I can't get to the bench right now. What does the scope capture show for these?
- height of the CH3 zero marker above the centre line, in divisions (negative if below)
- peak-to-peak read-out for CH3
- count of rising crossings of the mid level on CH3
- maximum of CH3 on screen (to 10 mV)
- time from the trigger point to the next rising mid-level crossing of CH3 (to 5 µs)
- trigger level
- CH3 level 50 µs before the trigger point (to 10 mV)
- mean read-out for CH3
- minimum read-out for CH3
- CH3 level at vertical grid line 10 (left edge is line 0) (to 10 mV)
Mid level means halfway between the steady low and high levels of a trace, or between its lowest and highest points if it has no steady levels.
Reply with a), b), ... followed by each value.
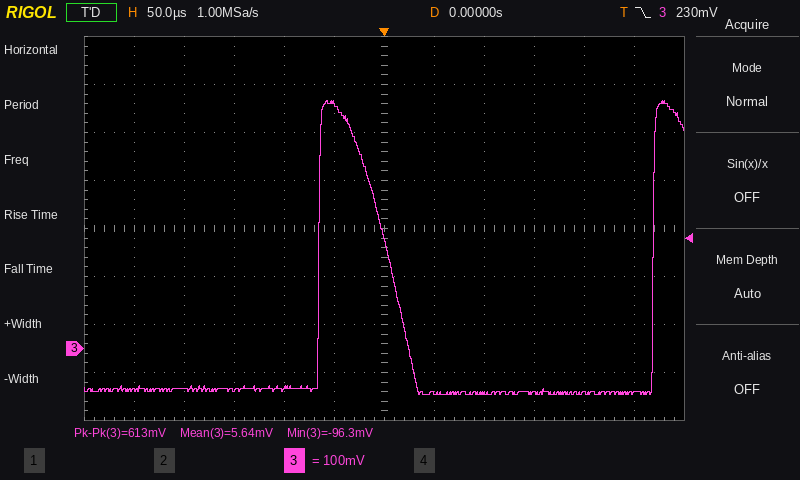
a) -2.5 div
b) 613 mV
c) 2
d) 520 mV
e) 270 µs
f) 230 mV
g) 510 mV
h) 5.64 mV
i) -96.3 mV
j) -90 mV
